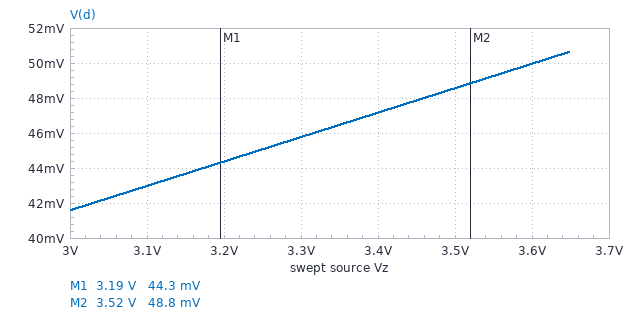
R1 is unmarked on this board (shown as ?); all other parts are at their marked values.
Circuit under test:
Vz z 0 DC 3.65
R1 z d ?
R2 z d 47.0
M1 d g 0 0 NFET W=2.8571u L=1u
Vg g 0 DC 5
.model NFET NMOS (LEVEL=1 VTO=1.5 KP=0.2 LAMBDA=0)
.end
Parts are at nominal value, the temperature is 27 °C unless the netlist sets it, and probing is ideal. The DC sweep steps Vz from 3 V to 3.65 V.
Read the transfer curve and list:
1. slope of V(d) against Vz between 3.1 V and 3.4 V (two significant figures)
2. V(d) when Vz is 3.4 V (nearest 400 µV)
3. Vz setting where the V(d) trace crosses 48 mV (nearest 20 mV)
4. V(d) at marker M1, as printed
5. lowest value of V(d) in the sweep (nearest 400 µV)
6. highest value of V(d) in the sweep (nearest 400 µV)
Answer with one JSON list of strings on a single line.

["0.014 V/V", "47.2 mV", "3.46 V", "44.3 mV", "41.6 mV", "50.8 mV"]
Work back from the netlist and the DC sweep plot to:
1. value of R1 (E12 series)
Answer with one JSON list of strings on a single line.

["150 Ω"]
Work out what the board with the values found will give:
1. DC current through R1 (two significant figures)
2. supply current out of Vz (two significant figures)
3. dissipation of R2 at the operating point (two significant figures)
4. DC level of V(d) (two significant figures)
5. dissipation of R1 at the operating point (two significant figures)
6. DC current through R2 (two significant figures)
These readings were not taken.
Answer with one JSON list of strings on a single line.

["24 mA", "100 mA", "280 mW", "51 mV", "86 mW", "77 mA"]
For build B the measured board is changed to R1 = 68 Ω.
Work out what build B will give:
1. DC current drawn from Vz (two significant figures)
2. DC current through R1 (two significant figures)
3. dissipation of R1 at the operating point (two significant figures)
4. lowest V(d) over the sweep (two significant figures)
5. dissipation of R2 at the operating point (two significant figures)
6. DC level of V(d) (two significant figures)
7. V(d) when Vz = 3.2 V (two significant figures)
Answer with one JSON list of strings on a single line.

["130 mA", "53 mA", "190 mW", "53 mV", "270 mW", "65 mV", "57 mV"]
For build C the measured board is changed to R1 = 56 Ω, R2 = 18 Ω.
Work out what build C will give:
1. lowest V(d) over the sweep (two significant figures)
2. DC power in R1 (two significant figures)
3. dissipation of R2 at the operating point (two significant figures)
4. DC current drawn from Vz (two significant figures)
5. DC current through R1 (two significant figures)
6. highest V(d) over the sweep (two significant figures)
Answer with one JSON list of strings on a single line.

["110 mV", "220 mW", "690 mW", "260 mA", "63 mA", "130 mV"]
